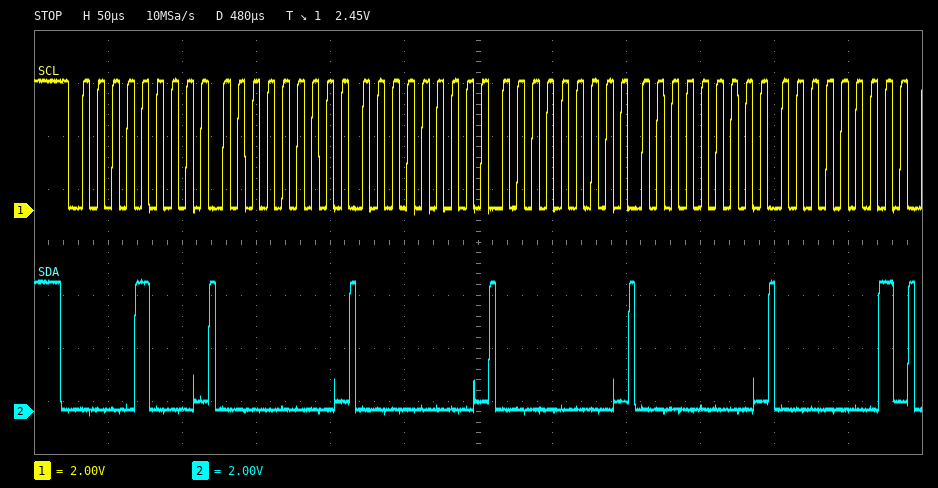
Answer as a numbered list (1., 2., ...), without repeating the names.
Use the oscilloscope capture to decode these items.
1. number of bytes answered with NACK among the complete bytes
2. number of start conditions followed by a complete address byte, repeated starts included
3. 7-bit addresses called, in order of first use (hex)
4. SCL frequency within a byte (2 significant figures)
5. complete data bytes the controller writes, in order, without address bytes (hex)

1. 0
2. 1
3. 0x04
4. 100 kHz
5. 00 00 00 00 01
